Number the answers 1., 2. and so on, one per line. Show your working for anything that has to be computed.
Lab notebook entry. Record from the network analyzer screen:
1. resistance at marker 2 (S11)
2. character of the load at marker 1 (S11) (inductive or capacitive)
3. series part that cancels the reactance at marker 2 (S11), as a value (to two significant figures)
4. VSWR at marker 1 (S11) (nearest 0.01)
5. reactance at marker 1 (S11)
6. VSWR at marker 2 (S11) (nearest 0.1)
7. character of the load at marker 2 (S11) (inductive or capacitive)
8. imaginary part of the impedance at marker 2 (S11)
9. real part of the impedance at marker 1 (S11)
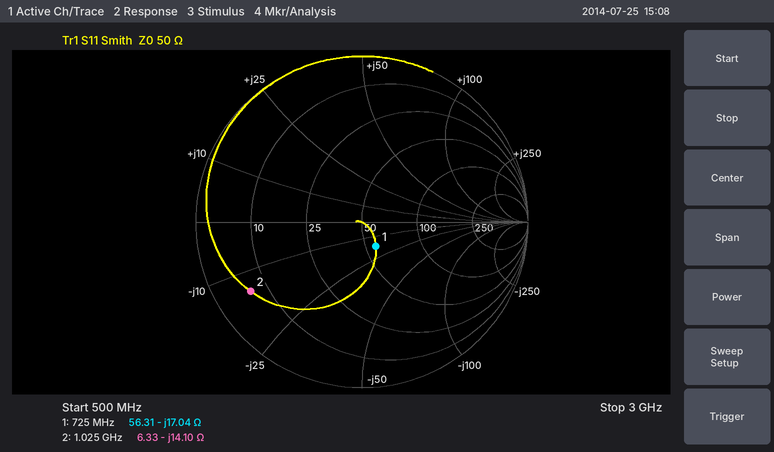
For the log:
1. 6.33 Ω
2. capacitive
3. L = 14.1 Ω/(2π × 1.025 GHz) ≈ 2.2 nH
4. 1.41
5. -17.04 Ω
6. 8.5
7. capacitive
8. -14.10 Ω
9. 56.31 Ω
